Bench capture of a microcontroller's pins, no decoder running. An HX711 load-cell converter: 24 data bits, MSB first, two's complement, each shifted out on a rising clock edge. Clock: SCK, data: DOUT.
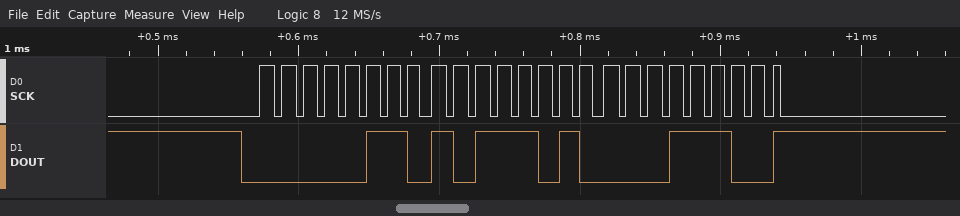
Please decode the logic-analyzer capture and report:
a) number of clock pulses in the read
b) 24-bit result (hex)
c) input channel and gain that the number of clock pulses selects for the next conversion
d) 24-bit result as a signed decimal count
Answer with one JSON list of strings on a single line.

["25", "0x06BA1C", "channel A, gain 128", "440860"]
